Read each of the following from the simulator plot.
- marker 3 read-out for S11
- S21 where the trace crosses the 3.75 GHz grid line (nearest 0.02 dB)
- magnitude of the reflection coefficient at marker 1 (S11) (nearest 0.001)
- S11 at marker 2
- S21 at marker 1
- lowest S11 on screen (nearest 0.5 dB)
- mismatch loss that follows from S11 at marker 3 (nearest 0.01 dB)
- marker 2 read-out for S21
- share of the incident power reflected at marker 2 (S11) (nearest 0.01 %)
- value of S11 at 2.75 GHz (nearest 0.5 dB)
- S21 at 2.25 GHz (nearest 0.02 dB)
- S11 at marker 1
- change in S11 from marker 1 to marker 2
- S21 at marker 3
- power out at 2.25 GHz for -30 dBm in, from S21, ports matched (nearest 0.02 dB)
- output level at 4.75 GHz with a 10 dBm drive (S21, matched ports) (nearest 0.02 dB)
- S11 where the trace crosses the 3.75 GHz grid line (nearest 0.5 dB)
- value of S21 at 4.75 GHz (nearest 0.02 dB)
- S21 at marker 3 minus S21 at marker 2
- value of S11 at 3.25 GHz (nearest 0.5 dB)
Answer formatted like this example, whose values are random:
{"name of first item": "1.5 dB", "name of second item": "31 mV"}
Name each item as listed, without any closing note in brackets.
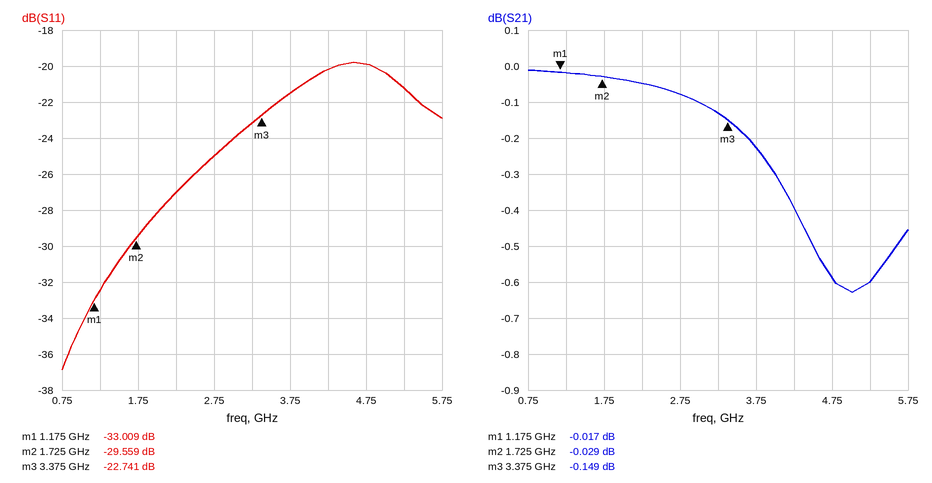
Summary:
{"marker 3 read-out for S11": "-22.741 dB", "S21 where the trace crosses the 3.75 GHz grid line": "-0.22 dB", "magnitude of the reflection coefficient at marker 1 (S11)": "0.022", "S11 at marker 2": "-29.559 dB", "S21 at marker 1": "-0.017 dB", "lowest S11 on screen": "-37.0 dB", "mismatch loss that follows from S11 at marker 3": "0.02 dB", "marker 2 read-out for S21": "-0.029 dB", "share of the incident power reflected at marker 2 (S11)": "0.11 %", "value of S11 at 2.75 GHz": "-25.0 dB", "S21 at 2.25 GHz": "-0.04 dB", "S11 at marker 1": "-33.009 dB", "change in S11 from marker 1 to marker 2": "3.450 dB", "S21 at marker 3": "-0.149 dB", "power out at 2.25 GHz for -30 dBm in, from S21, ports matched": "-30.04 dBm", "output level at 4.75 GHz with a 10 dBm drive (S21, matched ports)": "9.42 dBm", "S11 where the trace crosses the 3.75 GHz grid line": "-21.5 dB", "value of S21 at 4.75 GHz": "-0.58 dB", "S21 at marker 3 minus S21 at marker 2": "-0.120 dB", "value of S11 at 3.25 GHz": "-23.0 dB"}
